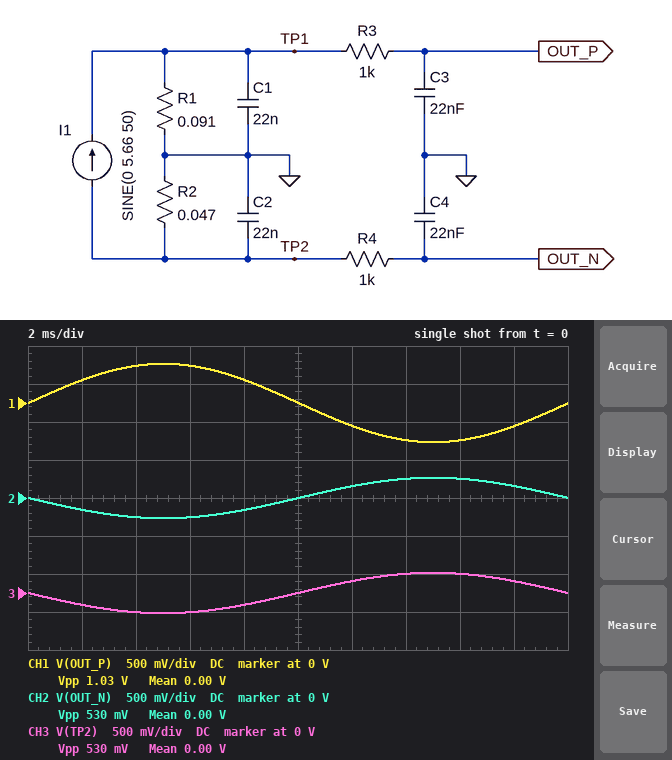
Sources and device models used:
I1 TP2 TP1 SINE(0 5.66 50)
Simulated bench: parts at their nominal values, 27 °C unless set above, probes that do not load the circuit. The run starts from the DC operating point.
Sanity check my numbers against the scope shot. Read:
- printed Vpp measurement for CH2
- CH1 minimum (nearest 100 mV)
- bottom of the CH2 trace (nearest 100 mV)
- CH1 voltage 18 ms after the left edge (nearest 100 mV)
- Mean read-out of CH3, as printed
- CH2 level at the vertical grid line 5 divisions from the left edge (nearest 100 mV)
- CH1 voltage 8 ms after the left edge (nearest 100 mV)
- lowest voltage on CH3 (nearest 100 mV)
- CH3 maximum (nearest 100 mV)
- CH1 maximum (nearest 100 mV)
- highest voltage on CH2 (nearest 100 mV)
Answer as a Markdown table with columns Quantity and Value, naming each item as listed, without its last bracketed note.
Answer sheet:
| Quantity | Value |
|---|---|
| printed Vpp measurement for CH2 | 530 mV |
| CH1 minimum | -500 mV |
| bottom of the CH2 trace | -300 mV |
| CH1 voltage 18 ms after the left edge | -300 mV |
| Mean read-out of CH3, as printed | 0.00 V |
| CH2 level at the vertical grid line 5 divisions from the left edge | 0 V |
| CH1 voltage 8 ms after the left edge | 300 mV |
| lowest voltage on CH3 | -300 mV |
| CH3 maximum | 300 mV |
| CH1 maximum | 500 mV |
| highest voltage on CH2 | 300 mV |
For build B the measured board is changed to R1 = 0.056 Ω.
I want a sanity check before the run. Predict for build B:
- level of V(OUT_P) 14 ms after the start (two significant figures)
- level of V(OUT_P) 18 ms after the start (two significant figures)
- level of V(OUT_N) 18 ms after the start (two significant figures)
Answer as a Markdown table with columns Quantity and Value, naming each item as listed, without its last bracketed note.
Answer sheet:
| Quantity | Value |
|---|---|
| level of V(OUT_P) 14 ms after the start | -300 mV |
| level of V(OUT_P) 18 ms after the start | -190 mV |
| level of V(OUT_N) 18 ms after the start | 160 mV |
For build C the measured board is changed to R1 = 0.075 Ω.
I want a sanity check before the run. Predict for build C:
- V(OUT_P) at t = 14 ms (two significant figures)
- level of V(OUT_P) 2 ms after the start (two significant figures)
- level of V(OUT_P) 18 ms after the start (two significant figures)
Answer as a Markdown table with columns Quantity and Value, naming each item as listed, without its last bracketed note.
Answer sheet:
| Quantity | Value |
|---|---|
| V(OUT_P) at t = 14 ms | -400 mV |
| level of V(OUT_P) 2 ms after the start | 250 mV |
| level of V(OUT_P) 18 ms after the start | -250 mV |
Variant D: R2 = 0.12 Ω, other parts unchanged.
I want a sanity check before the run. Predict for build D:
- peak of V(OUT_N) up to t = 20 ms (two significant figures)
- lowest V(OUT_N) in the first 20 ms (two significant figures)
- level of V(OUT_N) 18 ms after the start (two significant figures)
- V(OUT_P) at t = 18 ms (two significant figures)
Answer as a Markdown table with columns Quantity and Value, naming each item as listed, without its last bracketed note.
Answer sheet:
| Quantity | Value |
|---|---|
| peak of V(OUT_N) up to t = 20 ms | 680 mV |
| lowest V(OUT_N) in the first 20 ms | -680 mV |
| level of V(OUT_N) 18 ms after the start | 400 mV |
| V(OUT_P) at t = 18 ms | -310 mV |
